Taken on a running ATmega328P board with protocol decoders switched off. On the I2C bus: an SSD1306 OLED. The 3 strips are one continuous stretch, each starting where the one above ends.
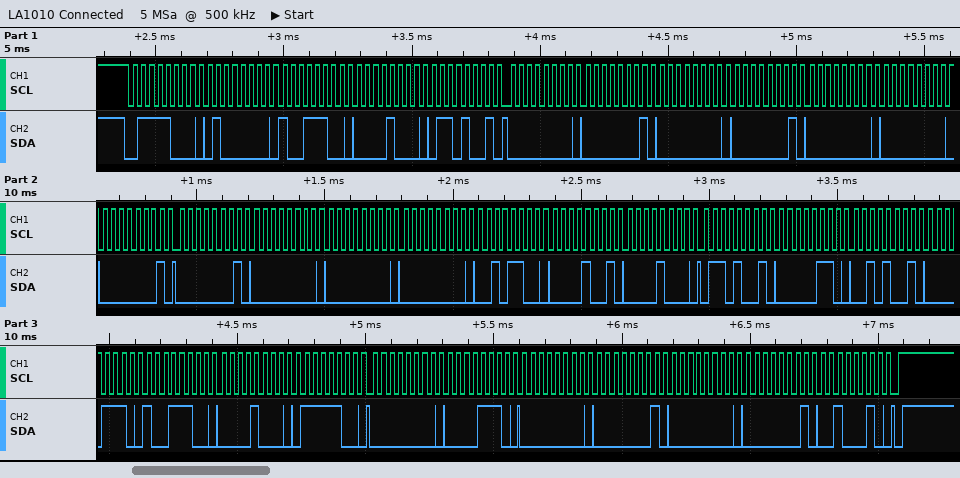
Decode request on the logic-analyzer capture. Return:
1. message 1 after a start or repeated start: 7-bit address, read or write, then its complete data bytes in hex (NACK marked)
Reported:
0x3C write: 40 9C 08 69 00 01 00 01 00 00 01 01 00 00 00 2C 09 08 69 06 29 0E 9C 08 7C 00 0E 00 01 00 01 22
